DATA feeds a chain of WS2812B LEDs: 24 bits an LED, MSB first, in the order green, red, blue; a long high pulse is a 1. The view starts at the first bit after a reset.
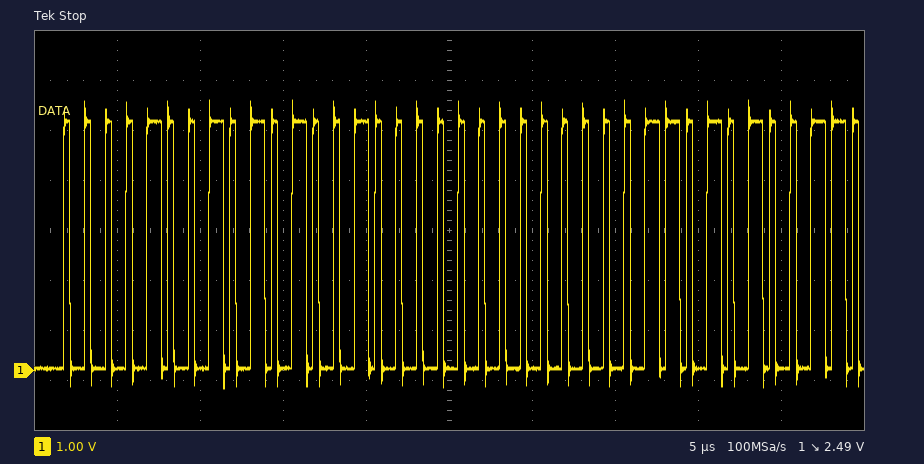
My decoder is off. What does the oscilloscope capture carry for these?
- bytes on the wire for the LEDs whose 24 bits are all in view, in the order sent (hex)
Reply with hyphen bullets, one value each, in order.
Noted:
- 09 52 00
